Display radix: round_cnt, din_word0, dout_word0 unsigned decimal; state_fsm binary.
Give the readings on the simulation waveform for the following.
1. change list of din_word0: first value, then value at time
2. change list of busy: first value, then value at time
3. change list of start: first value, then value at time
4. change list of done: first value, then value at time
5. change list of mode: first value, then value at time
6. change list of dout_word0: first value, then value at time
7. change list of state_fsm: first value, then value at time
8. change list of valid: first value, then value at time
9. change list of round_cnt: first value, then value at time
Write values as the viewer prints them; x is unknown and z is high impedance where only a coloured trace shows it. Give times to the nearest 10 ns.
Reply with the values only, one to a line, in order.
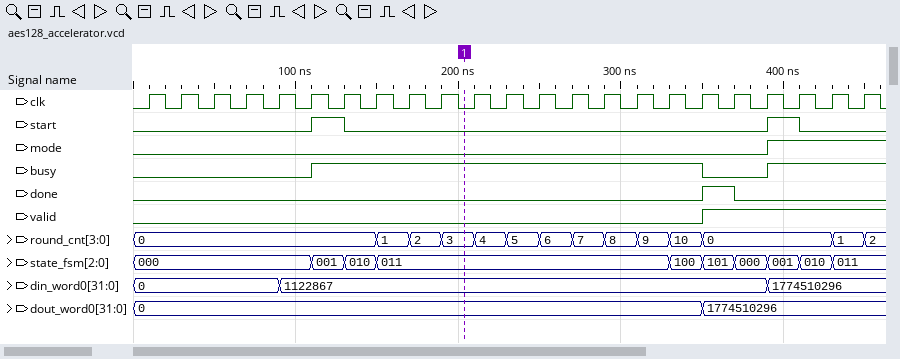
0, 1122867 at 90 ns, 1774510296 at 390 ns
0, 1 at 110 ns, 0 at 350 ns, 1 at 390 ns
0, 1 at 110 ns, 0 at 130 ns, 1 at 390 ns, 0 at 410 ns
0, 1 at 350 ns, 0 at 370 ns
0, 1 at 390 ns
0, 1774510296 at 350 ns
000, 001 at 110 ns, 010 at 130 ns, 011 at 150 ns, 100 at 330 ns, 101 at 350 ns, 000 at 370 ns, 001 at 390 ns, 010 at 410 ns, 011 at 430 ns
0, 1 at 350 ns
0, 1 at 150 ns, 2 at 170 ns, 3 at 190 ns, 4 at 210 ns, 5 at 230 ns, 6 at 250 ns, 7 at 270 ns, 8 at 290 ns, 9 at 310 ns, 10 at 330 ns, 0 at 350 ns, 1 at 430 ns, 2 at 450 ns
